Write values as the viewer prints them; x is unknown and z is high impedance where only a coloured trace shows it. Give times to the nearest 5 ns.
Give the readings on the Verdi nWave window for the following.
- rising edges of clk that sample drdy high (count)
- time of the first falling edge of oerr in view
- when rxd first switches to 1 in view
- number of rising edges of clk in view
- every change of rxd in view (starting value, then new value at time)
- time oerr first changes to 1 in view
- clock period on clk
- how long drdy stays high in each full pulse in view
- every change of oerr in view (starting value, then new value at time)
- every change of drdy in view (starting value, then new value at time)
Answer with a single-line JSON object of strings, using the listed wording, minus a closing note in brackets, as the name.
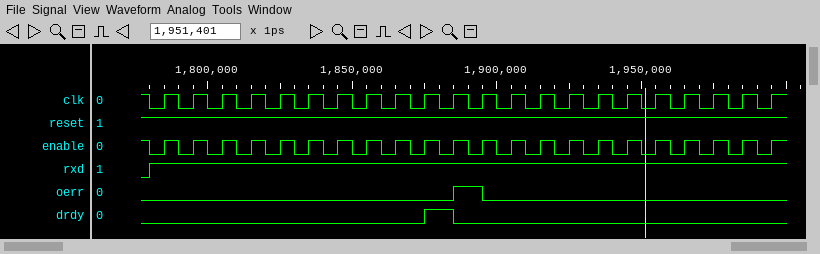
{"rising edges of clk that sample drdy high": "1", "time of the first falling edge of oerr in view": "1895 ns", "when rxd first switches to 1 in view": "1780 ns", "number of rising edges of clk in view": "22", "every change of rxd in view": "0, 1 at 1780 ns", "time oerr first changes to 1 in view": "1885 ns", "clock period on clk": "10 ns", "how long drdy stays high in each full pulse in view": "10 ns", "every change of oerr in view": "0, 1 at 1885 ns, 0 at 1895 ns", "every change of drdy in view": "0, 1 at 1875 ns, 0 at 1885 ns"}
